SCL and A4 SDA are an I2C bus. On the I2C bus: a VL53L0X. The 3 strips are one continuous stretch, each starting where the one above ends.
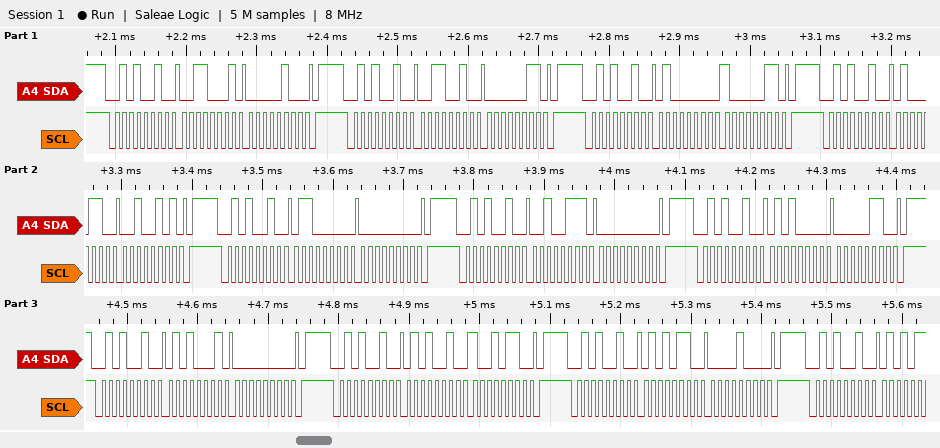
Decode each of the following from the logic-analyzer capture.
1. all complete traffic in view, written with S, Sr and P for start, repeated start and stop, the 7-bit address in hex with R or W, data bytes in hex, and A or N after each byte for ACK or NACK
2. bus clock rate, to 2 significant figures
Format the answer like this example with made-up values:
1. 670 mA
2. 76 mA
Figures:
1. S 29W A 31 A 04 A P S 29W A 32 A 03 A P S 29W A 40 A 83 A P S 29W A 46 A 25 A P S 29W A 60 A 00 A P S 29W A 27 A 00 A P S 29W A 50 A 06 A P S 29W A 51 A 00 A P S 29W A 52 A 96 A P S 29W A 56 A 08 A P S 29W A
2. 100 kHz
